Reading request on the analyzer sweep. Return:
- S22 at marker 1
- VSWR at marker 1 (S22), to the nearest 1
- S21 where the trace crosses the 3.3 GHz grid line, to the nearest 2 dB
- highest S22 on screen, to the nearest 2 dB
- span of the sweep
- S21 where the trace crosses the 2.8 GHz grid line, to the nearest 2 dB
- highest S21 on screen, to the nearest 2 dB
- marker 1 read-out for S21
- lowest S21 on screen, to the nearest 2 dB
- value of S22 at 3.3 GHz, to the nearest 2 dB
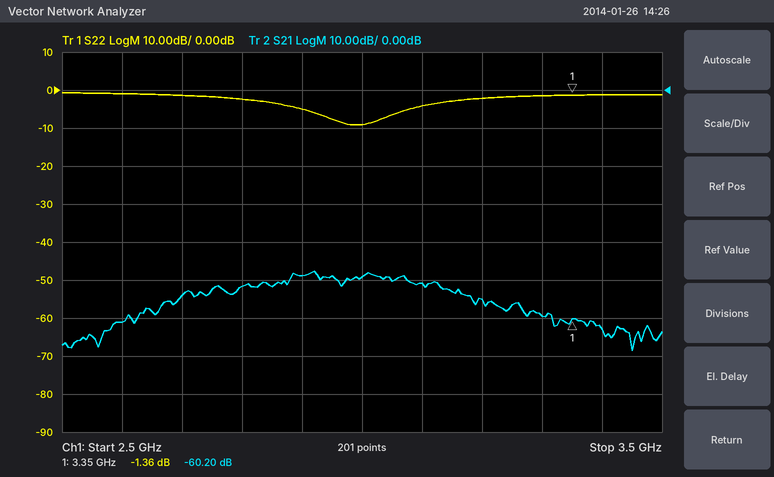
-1.36 dB
13
-60 dB
0 dB
1 GHz
-52 dB
-48 dB
-60.20 dB
-68 dB
-2 dB
